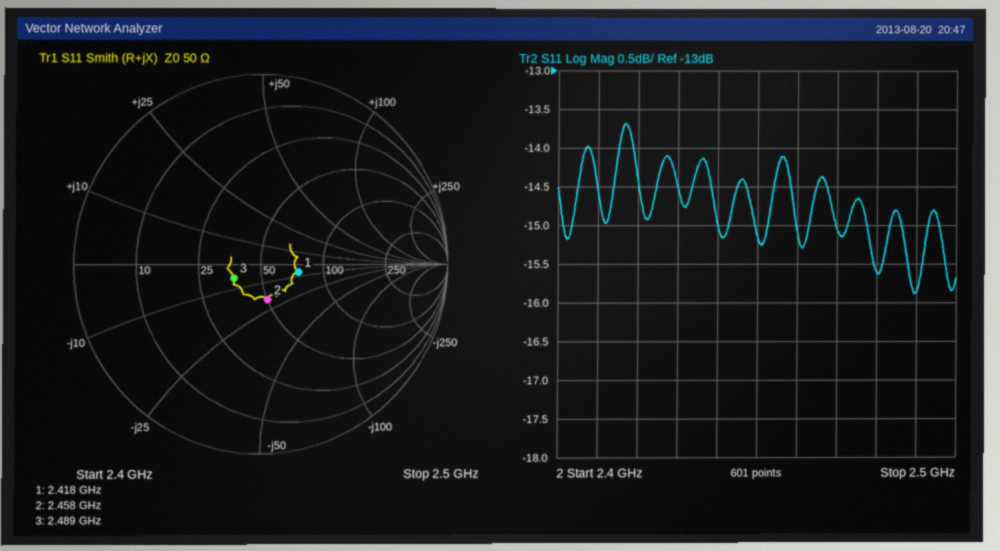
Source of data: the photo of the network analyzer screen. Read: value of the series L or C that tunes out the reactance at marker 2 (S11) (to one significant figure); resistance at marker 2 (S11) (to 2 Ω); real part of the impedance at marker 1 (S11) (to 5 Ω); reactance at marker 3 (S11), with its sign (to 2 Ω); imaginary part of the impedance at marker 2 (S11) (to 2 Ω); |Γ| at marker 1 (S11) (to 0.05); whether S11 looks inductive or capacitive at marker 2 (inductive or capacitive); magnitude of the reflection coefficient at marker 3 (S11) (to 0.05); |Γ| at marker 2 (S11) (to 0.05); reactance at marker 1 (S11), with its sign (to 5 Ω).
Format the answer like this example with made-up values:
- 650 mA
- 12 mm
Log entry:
- 1 nH
- 50 Ω
- 75 Ω
- -6 Ω
- -20 Ω
- 0.20
- capacitive
- 0.15
- 0.20
- -5 Ω
